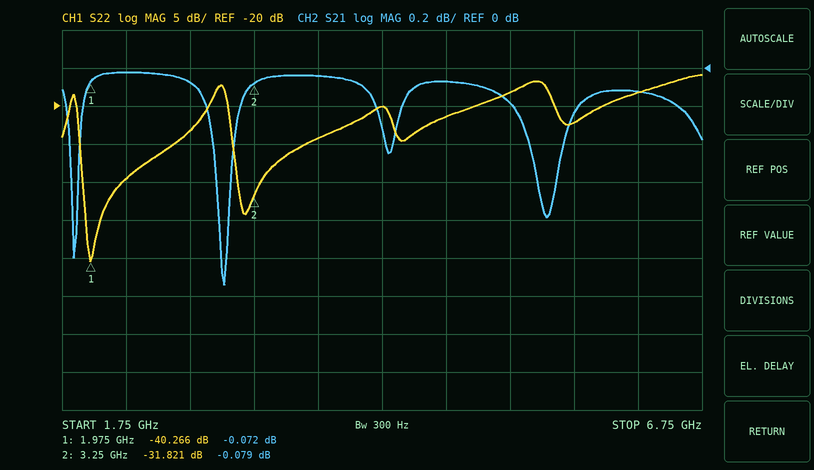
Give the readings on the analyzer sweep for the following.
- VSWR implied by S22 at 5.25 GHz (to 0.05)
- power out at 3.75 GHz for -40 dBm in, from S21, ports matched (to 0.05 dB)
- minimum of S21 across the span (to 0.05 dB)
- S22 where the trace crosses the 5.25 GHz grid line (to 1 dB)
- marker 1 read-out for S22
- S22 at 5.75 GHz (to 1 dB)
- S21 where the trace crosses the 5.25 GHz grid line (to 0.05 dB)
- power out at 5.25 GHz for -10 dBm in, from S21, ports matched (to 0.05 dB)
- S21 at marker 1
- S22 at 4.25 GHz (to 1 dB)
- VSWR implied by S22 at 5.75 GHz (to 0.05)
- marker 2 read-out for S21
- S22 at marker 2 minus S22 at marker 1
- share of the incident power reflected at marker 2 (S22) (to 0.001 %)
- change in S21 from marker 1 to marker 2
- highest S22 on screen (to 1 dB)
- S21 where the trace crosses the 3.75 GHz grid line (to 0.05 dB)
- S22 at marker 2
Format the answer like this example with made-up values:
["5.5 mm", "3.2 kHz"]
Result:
["1.30", "-40.05 dBm", "-1.15 dB", "-18 dB", "-40.266 dB", "-22 dB", "-0.20 dB", "-10.20 dBm", "-0.072 dB", "-20 dB", "1.15", "-0.079 dB", "8.445 dB", "0.066 %", "-0.007 dB", "-16 dB", "-0.05 dB", "-31.821 dB"]
